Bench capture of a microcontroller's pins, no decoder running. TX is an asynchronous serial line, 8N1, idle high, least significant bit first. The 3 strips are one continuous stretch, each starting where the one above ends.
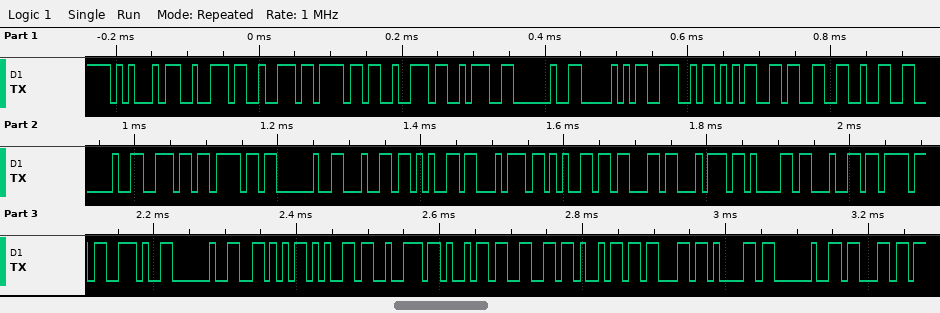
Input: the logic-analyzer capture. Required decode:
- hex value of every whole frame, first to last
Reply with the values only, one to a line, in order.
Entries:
45 72 72 6F 72 3A 20 50 4E 35 33 32 20 6E 6F 20 64 65 74 65 63 74 61 64 6F 2E 20 56 65 72 69 66 69 63 61 20 63
